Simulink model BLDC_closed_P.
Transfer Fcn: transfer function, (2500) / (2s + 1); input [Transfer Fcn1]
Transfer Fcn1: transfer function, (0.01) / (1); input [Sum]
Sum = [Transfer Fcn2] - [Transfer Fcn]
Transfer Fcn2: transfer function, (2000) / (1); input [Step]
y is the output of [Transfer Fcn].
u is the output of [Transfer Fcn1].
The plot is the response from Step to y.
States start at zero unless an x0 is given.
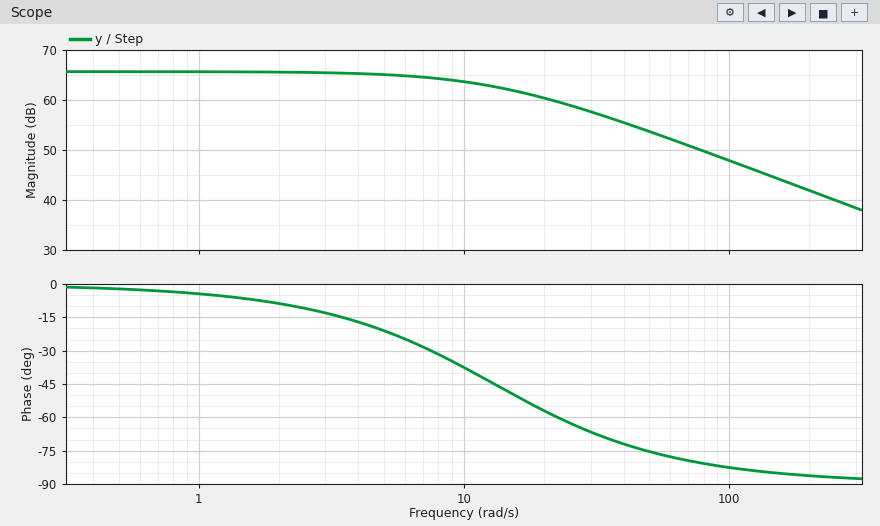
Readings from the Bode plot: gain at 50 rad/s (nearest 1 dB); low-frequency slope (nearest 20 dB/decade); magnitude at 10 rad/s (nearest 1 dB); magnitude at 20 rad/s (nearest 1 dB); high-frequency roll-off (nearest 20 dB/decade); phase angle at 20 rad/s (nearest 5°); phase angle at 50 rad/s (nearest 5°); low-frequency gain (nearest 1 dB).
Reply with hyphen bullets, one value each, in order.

- 54 dB
- 0 dB/decade
- 64 dB
- 60 dB
- -20 dB/decade
- -55°
- -75°
- 66 dB
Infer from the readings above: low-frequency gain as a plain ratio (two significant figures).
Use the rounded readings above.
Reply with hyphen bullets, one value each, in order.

- 2000
